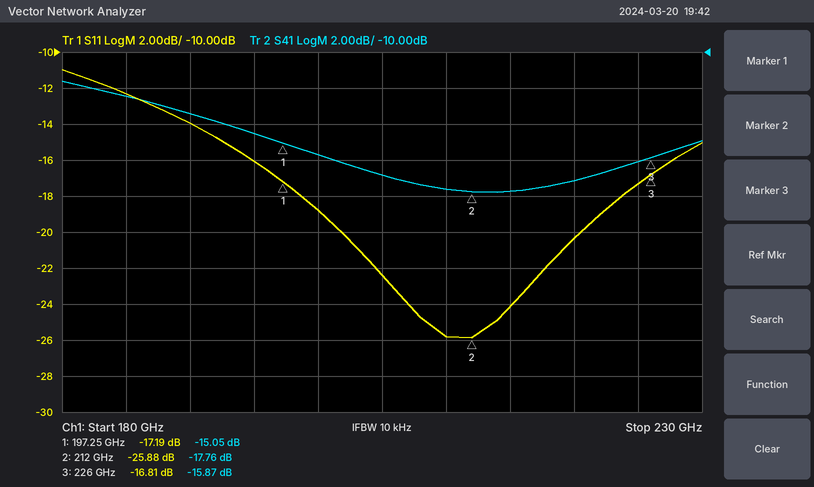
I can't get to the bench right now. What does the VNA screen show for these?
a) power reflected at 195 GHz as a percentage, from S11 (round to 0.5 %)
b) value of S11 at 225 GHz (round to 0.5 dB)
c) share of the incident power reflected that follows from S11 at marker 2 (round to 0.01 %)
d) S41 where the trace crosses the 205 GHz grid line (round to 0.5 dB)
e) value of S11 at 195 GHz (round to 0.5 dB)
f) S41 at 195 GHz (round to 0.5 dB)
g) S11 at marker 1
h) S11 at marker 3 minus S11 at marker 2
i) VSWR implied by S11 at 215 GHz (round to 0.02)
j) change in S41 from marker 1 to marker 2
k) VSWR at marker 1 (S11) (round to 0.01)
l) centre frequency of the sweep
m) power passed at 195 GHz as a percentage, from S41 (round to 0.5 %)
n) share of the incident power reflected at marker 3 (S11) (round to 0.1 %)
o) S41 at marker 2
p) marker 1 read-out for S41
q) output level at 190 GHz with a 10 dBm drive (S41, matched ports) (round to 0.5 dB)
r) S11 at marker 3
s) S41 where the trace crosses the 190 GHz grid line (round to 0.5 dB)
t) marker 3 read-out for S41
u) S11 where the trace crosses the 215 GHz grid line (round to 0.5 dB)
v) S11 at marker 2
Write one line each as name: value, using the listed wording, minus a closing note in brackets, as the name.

power reflected at 195 GHz as a percentage, from S11: 2.5 %
value of S11 at 225 GHz: -17.5 dB
share of the incident power reflected that follows from S11 at marker 2: 0.26 %
S41 where the trace crosses the 205 GHz grid line: -17.0 dB
value of S11 at 195 GHz: -16.0 dB
S41 at 195 GHz: -14.5 dB
S11 at marker 1: -17.19 dB
S11 at marker 3 minus S11 at marker 2: 9.07 dB
VSWR implied by S11 at 215 GHz: 1.14
change in S41 from marker 1 to marker 2: -2.71 dB
VSWR at marker 1 (S11): 1.32
centre frequency of the sweep: 205 GHz
power passed at 195 GHz as a percentage, from S41: 3.5 %
share of the incident power reflected at marker 3 (S11): 2.1 %
S41 at marker 2: -17.76 dB
marker 1 read-out for S41: -15.05 dB
output level at 190 GHz with a 10 dBm drive (S41, matched ports): -3.5 dBm
S11 at marker 3: -16.81 dB
S41 where the trace crosses the 190 GHz grid line: -13.5 dB
marker 3 read-out for S41: -15.87 dB
S11 where the trace crosses the 215 GHz grid line: -24.0 dB
S11 at marker 2: -25.88 dB
